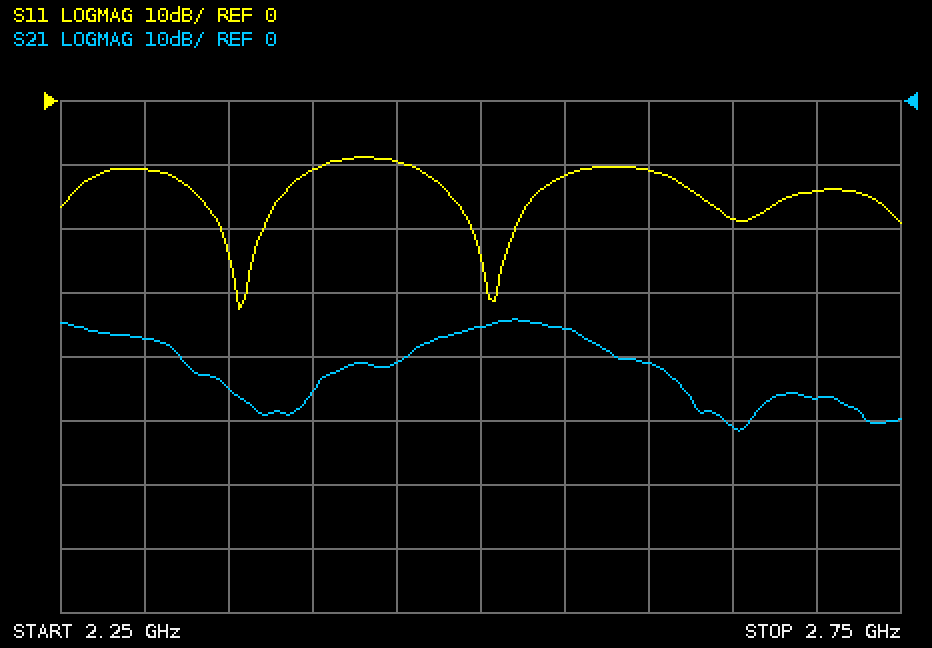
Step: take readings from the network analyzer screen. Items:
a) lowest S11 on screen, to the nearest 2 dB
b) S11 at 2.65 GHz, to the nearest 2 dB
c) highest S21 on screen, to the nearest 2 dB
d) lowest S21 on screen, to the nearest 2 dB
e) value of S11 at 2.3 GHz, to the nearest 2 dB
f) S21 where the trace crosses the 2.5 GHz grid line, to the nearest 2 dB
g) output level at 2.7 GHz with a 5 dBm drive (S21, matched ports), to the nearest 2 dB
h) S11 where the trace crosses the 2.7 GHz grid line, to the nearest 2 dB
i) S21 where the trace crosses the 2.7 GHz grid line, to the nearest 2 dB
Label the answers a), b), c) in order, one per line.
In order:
a) -32 dB
b) -18 dB
c) -34 dB
d) -52 dB
e) -10 dB
f) -36 dB
g) -42 dBm
h) -14 dB
i) -46 dB
